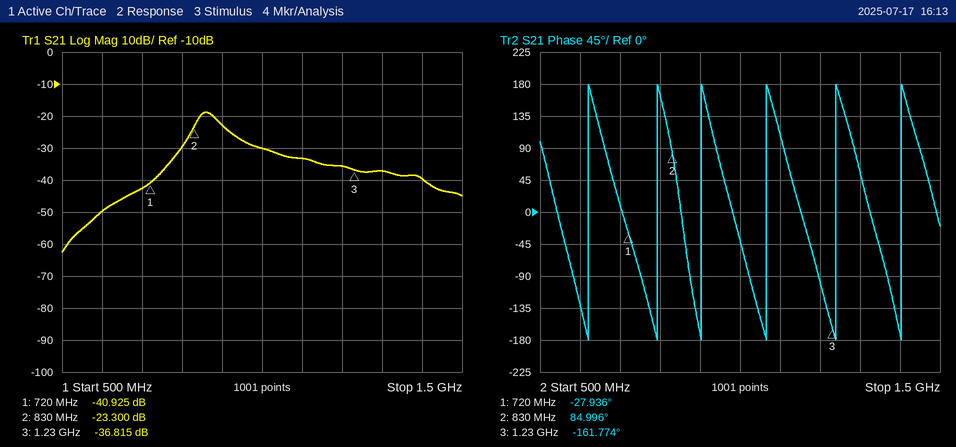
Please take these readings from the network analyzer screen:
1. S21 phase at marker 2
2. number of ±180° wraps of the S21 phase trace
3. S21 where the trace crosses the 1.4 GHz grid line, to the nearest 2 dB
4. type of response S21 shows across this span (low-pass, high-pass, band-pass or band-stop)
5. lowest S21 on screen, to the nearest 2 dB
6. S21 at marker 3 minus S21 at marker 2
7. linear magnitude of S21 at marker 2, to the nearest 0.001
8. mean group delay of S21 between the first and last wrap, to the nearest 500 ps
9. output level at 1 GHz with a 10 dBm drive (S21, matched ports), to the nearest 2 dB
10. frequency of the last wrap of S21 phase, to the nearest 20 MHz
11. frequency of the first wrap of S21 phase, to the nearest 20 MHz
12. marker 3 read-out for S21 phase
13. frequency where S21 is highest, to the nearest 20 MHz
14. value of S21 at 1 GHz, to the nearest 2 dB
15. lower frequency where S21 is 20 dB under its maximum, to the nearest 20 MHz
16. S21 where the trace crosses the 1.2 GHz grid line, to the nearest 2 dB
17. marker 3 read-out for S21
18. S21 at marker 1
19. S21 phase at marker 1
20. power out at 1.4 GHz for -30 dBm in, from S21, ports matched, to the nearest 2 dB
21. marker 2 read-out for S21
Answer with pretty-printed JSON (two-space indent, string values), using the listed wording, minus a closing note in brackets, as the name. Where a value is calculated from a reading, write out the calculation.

{
  "S21 phase at marker 2": "84.996°",
  "number of ±180° wraps of the S21 phase trace": "6",
  "S21 where the trace crosses the 1.4 GHz grid line, to the nearest 2 dB": "-40 dB",
  "type of response S21 shows across this span": "band-pass",
  "lowest S21 on screen, to the nearest 2 dB": "-62 dB",
  "S21 at marker 3 minus S21 at marker 2": "-36.815 − (-23.3) = -13.515 dB",
  "linear magnitude of S21 at marker 2, to the nearest 0.001": "10^(-23.3/20) ≈ 0.068",
  "mean group delay of S21 between the first and last wrap, to the nearest 500 ps": "5 cycles / (1.40 GHz − 620 MHz) ≈ 6.41 ns, so 6.5 ns to the nearest 500 ps",
  "output level at 1 GHz with a 10 dBm drive (S21, matched ports), to the nearest 2 dB": "10 dBm + (-30 dB) = -20 dBm",
  "frequency of the last wrap of S21 phase, to the nearest 20 MHz": "1.40 GHz",
  "frequency of the first wrap of S21 phase, to the nearest 20 MHz": "620 MHz",
  "marker 3 read-out for S21 phase": "-161.774°",
  "frequency where S21 is highest, to the nearest 20 MHz": "860 MHz",
  "value of S21 at 1 GHz, to the nearest 2 dB": "-30 dB",
  "lower frequency where S21 is 20 dB under its maximum, to the nearest 20 MHz": "740 MHz",
  "S21 where the trace crosses the 1.2 GHz grid line, to the nearest 2 dB": "-36 dB",
  "marker 3 read-out for S21": "-36.815 dB",
  "S21 at marker 1": "-40.925 dB",
  "S21 phase at marker 1": "-27.936°",
  "power out at 1.4 GHz for -30 dBm in, from S21, ports matched, to the nearest 2 dB": "-30 dBm + (-40 dB) = -70 dBm",
  "marker 2 read-out for S21": "-23.300 dB"
}
